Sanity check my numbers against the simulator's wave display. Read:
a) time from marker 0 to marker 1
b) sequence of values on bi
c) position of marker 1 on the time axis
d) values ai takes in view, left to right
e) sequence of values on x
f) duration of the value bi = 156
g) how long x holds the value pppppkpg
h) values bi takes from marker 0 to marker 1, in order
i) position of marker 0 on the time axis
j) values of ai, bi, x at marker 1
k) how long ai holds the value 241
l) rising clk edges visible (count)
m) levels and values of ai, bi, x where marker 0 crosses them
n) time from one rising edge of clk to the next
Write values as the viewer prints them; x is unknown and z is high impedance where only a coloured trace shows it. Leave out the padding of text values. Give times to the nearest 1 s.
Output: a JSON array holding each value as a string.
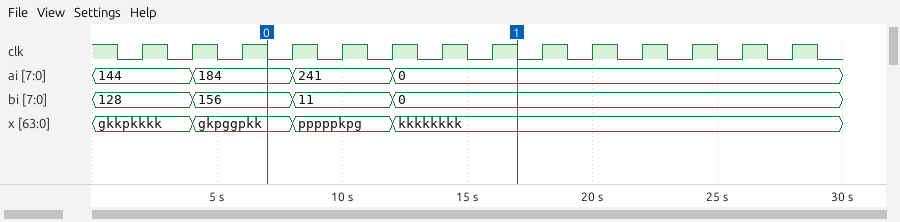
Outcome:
["10 s", "128, 156, 11, 0", "17 s", "144, 184, 241, 0", "gkkpkkkk, gkpggpkk, pppppkpg, kkkkkkkk", "4 s", "4 s", "156, 11, 0", "7 s", "ai=0, bi=0, x=kkkkkkkk", "4 s", "14", "ai=184, bi=156, x=gkpggpkk", "2 s"]
